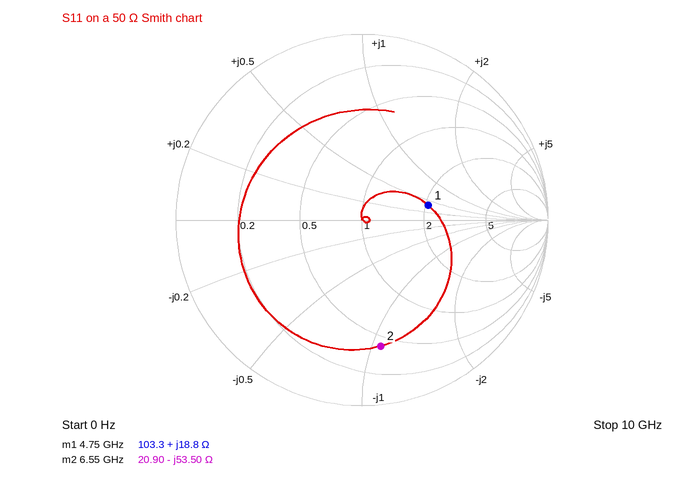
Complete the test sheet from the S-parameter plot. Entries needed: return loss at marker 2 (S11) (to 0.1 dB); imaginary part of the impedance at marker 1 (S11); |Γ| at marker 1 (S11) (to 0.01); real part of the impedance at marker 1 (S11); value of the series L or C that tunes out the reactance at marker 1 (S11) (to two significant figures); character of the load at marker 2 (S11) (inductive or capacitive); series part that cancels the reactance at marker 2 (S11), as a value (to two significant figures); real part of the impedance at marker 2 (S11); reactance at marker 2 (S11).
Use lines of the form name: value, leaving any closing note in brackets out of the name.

return loss at marker 2 (S11): 3.3 dB
imaginary part of the impedance at marker 1: +18.8 Ω
|Γ| at marker 1 (S11): 0.37
real part of the impedance at marker 1: 103.3 Ω
value of the series L or C that tunes out the reactance at marker 1 (S11): 1.8 pF
character of the load at marker 2 (S11): capacitive
series part that cancels the reactance at marker 2 (S11), as a value: 1.3 nH
real part of the impedance at marker 2: 20.90 Ω
reactance at marker 2: -53.50 Ω
